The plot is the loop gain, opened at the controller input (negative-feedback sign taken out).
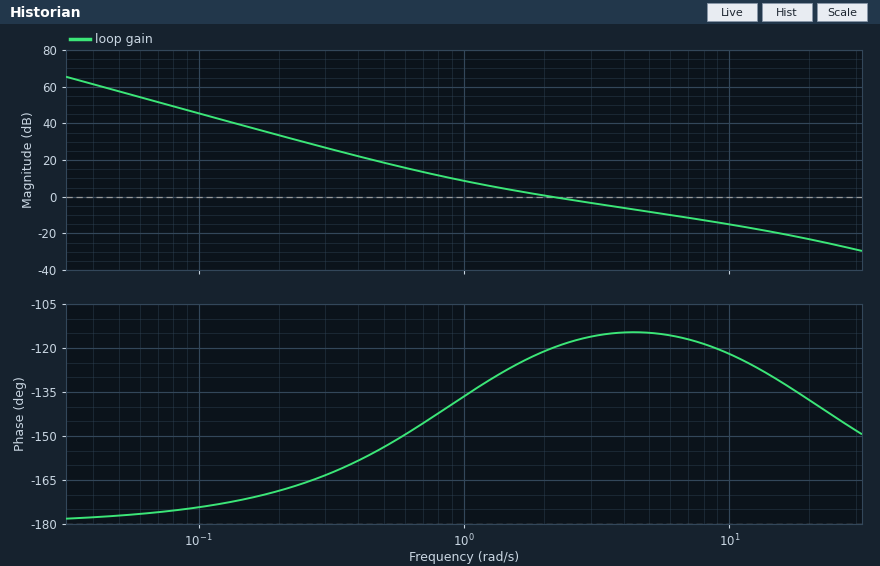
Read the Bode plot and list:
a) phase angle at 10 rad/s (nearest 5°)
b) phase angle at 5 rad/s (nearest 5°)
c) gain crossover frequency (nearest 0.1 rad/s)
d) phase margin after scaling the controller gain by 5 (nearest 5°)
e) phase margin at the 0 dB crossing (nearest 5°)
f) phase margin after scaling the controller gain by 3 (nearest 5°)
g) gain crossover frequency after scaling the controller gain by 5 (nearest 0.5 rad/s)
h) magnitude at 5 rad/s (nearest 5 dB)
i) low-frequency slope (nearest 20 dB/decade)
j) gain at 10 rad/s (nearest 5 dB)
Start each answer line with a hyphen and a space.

- -120°
- -115°
- 2.1 rad/s
- 60°
- 60°
- 65°
- 9.0 rad/s
- -10 dB
- -40 dB/decade
- -15 dB
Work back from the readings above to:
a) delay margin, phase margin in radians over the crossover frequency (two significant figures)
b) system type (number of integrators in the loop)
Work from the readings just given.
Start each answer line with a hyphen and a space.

- 0.50 s
- 2
